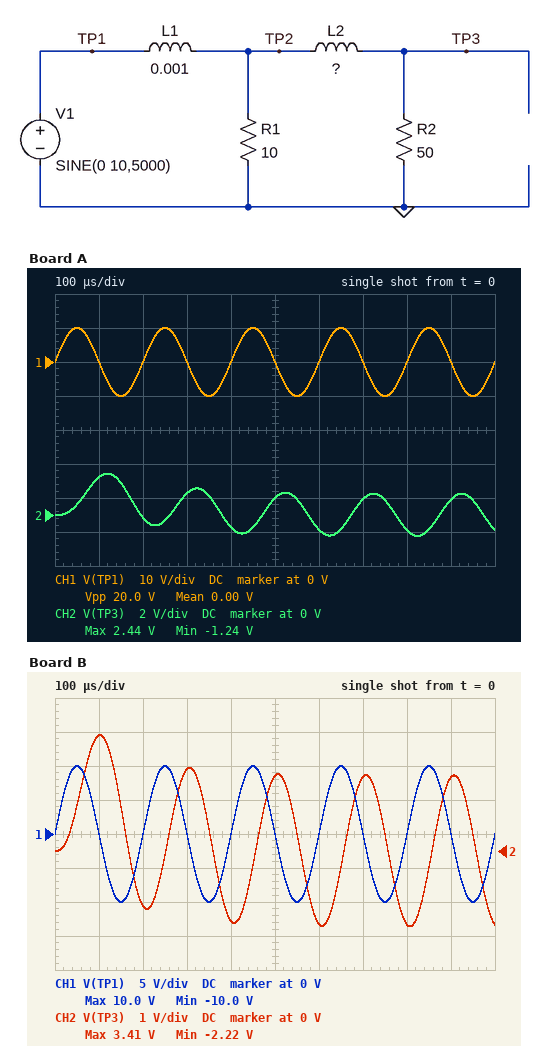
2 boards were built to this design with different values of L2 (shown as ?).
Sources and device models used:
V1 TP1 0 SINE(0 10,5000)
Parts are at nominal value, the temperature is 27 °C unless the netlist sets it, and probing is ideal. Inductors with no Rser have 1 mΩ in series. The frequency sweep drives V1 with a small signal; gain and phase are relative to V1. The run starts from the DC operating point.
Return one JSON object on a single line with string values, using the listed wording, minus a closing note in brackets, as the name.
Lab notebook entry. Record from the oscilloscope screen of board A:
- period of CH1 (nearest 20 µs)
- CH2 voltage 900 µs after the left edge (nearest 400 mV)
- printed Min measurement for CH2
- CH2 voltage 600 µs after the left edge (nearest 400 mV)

{"period of CH1": "200 µs", "CH2 voltage 900 µs after the left edge": "800 mV", "printed Min measurement for CH2": "-1.24 V", "CH2 voltage 600 µs after the left edge": "-800 mV"}
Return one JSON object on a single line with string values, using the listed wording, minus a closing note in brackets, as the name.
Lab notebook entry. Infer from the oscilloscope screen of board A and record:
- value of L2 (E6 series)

{"value of L2": "3.3 mH"}
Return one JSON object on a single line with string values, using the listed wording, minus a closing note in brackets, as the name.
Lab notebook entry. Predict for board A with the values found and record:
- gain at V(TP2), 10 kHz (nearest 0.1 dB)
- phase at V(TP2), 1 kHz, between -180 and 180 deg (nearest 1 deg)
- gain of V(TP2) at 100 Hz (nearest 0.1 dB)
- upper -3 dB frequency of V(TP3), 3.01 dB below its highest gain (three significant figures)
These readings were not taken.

{"gain at V(TP2), 10 kHz": "-16.2 dB", "phase at V(TP2), 1 kHz, between -180 and 180 deg": "-35 deg", "gain of V(TP2) at 100 Hz": "0 dB", "upper -3 dB frequency of V(TP3), 3.01 dB below its highest gain": "1.04 kHz"}
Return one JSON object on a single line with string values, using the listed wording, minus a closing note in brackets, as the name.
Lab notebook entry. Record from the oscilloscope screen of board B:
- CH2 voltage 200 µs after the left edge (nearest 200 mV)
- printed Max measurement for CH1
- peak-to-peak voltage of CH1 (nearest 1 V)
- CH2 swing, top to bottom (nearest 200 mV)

{"CH2 voltage 200 µs after the left edge": "-1.6 V", "printed Max measurement for CH1": "10.0 V", "peak-to-peak voltage of CH1": "20 V", "CH2 swing, top to bottom": "5.6 V"}
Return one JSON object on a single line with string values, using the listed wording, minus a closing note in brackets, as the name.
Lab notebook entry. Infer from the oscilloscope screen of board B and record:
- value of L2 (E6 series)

{"value of L2": "1 mH"}
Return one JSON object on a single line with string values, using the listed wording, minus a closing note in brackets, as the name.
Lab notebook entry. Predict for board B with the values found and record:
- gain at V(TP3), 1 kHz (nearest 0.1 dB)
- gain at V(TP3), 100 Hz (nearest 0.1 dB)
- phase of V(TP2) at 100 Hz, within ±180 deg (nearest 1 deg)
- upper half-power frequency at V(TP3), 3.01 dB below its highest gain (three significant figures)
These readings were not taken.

{"gain at V(TP3), 1 kHz": "-2.1 dB", "gain at V(TP3), 100 Hz": "0 dB", "phase of V(TP2) at 100 Hz, within ±180 deg": "-4 deg", "upper half-power frequency at V(TP3), 3.01 dB below its highest gain": "1.26 kHz"}
